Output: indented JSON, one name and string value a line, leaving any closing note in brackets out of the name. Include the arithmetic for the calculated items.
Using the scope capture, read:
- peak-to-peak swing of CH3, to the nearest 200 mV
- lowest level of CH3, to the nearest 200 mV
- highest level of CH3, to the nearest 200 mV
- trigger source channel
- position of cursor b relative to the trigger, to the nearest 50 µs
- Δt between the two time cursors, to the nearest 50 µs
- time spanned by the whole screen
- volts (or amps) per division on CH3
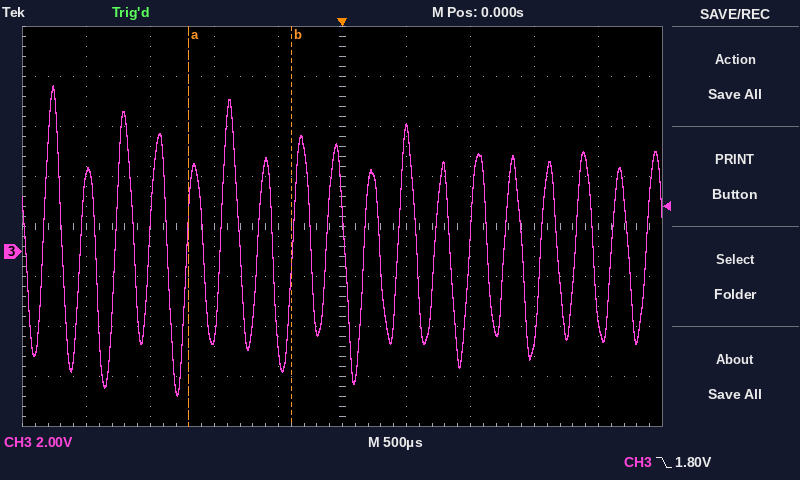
{
  "peak-to-peak swing of CH3, to the nearest 200 mV": "6.6 V − (-5.8 V) = 12.4 V",
  "lowest level of CH3, to the nearest 200 mV": "-5.8 V",
  "highest level of CH3, to the nearest 200 mV": "6.6 V",
  "trigger source channel": "CH3",
  "position of cursor b relative to the trigger, to the nearest 50 µs": "-400 µs",
  "Δt between the two time cursors, to the nearest 50 µs": "800 µs",
  "time spanned by the whole screen": "5 ms",
  "volts (or amps) per division on CH3": "2 V"
}
